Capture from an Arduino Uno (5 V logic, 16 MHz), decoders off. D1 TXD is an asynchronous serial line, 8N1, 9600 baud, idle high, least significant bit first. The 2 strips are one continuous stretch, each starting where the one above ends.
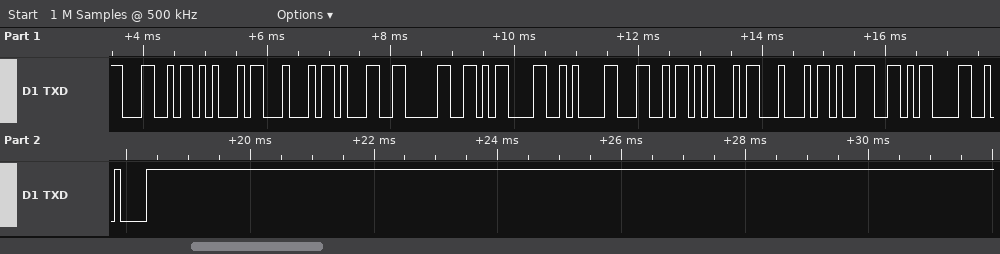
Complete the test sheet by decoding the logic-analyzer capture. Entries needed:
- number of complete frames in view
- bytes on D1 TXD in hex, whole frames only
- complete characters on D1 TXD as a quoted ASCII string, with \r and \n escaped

13
4C 45 44 31 30 0D 0A 4C 45 44 39 0D 0A
"LED10\r\nLED9\r\n"
